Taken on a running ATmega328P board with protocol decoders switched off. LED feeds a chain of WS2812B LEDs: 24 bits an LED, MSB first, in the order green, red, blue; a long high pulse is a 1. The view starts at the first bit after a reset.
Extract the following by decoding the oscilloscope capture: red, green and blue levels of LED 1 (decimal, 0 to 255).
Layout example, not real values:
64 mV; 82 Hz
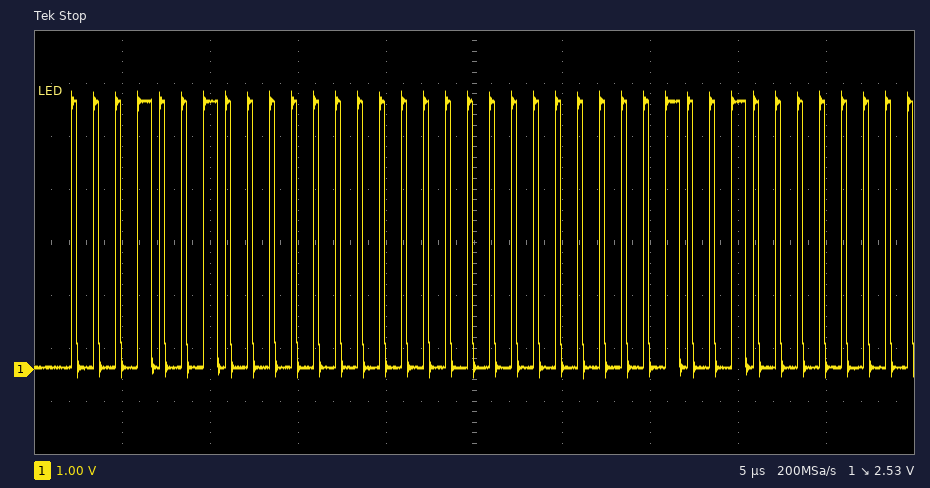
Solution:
0, 18, 0
